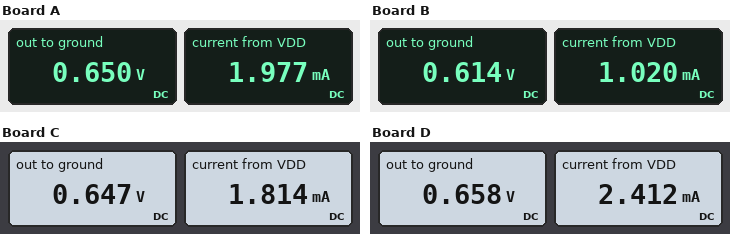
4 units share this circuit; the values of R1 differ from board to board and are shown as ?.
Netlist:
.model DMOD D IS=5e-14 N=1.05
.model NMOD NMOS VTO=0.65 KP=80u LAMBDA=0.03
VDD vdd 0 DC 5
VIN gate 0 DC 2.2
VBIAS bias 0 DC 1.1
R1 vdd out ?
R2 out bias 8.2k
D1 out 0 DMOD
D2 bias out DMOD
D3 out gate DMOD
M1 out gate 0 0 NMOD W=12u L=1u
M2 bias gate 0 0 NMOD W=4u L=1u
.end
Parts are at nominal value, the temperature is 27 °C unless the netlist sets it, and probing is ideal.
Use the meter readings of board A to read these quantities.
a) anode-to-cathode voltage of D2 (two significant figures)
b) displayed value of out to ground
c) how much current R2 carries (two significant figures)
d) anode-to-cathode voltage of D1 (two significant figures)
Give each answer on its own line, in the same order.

450 mV
0.650 V
55 µA
650 mV
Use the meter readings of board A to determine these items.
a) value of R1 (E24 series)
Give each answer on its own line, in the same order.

2.2 kΩ
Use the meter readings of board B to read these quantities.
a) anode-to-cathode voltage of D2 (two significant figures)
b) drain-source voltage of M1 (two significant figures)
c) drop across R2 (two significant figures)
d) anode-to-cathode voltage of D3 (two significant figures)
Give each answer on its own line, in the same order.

490 mV
610 mV
490 mV
-1.6 V
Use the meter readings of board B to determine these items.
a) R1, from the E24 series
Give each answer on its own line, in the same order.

4.3 kΩ
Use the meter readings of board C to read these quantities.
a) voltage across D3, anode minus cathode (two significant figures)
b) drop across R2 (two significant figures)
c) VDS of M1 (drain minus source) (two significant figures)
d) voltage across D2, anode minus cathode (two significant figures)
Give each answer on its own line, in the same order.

-1.6 V
450 mV
650 mV
450 mV
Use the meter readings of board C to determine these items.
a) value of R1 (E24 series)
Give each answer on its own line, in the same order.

2.4 kΩ
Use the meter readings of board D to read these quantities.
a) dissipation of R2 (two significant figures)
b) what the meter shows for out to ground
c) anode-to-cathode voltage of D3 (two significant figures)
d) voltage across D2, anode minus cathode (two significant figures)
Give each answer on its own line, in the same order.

24 µW
0.658 V
-1.5 V
440 mV
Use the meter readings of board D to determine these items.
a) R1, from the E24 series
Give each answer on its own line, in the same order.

1.8 kΩ
